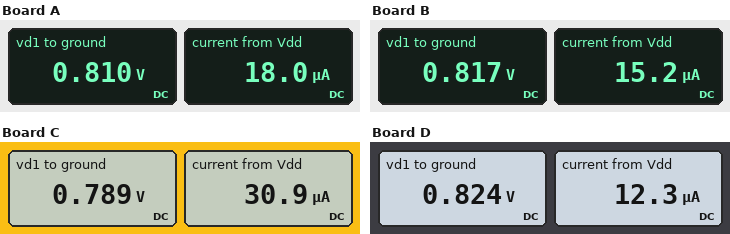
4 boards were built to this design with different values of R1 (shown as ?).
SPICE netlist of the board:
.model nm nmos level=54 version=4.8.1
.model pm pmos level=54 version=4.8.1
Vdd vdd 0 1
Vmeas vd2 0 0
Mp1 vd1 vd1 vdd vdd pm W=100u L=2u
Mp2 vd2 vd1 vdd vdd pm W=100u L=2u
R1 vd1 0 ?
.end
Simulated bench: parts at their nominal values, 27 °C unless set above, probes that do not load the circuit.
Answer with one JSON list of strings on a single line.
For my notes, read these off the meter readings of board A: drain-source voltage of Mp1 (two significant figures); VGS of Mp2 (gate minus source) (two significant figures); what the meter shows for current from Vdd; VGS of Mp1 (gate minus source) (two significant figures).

["-190 mV", "-190 mV", "18.0 µA", "-190 mV"]
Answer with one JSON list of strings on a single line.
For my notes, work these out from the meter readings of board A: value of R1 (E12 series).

["100 kΩ"]
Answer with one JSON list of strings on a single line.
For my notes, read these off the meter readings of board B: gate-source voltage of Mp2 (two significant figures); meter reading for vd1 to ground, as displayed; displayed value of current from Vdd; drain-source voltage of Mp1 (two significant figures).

["-180 mV", "0.817 V", "15.2 µA", "-180 mV"]
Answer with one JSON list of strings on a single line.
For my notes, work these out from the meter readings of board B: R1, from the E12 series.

["120 kΩ"]
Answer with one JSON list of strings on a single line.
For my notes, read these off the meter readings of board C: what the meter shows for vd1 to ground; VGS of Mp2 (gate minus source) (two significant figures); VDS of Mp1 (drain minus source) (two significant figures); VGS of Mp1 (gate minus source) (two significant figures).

["0.789 V", "-210 mV", "-210 mV", "-210 mV"]
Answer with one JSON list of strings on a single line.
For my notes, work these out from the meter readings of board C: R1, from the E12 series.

["56 kΩ"]
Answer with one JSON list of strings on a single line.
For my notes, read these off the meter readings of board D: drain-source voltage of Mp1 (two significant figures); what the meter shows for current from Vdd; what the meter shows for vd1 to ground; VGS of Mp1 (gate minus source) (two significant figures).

["-180 mV", "12.3 µA", "0.824 V", "-180 mV"]
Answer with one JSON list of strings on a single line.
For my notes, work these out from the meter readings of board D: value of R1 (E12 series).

["150 kΩ"]
